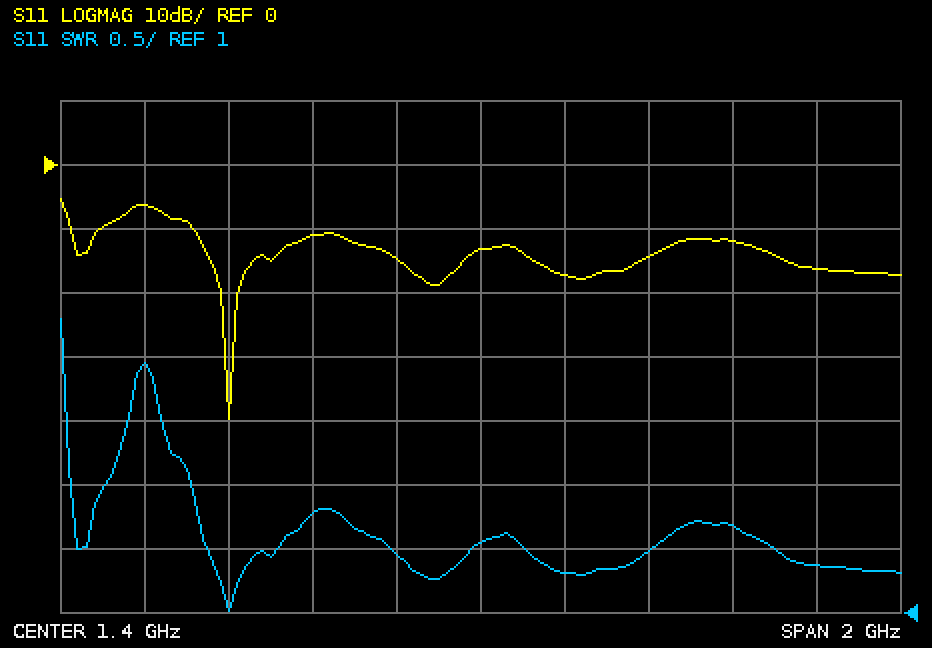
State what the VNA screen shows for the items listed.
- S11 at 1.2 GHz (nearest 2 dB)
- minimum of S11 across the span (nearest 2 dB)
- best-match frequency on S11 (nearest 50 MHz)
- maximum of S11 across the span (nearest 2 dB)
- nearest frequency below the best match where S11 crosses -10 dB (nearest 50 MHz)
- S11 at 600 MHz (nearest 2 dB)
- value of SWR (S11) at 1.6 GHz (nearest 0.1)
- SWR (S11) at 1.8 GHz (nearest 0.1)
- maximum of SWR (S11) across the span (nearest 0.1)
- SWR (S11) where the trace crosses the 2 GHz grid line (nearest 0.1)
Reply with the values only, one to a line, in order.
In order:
-14 dB
-40 dB
800 MHz
-6 dB
700 MHz
-6 dB
1.3
1.5
3.3
1.7
